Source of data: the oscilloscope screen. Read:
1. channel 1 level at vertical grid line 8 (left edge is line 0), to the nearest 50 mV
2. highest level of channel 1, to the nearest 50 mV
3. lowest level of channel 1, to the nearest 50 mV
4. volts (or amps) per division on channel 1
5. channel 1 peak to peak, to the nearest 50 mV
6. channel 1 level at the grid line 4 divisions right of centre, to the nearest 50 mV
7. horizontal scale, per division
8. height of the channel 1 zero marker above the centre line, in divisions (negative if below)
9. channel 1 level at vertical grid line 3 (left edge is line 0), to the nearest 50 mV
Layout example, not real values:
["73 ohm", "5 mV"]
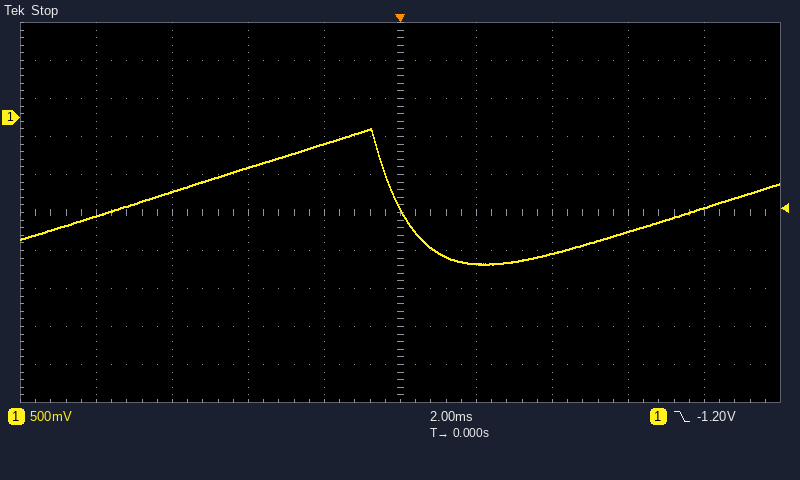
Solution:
["-1.50 V", "-150 mV", "-1.95 V", "500 mV", "1.80 V", "-1.20 V", "2 ms", "+2.5 div", "-650 mV"]
